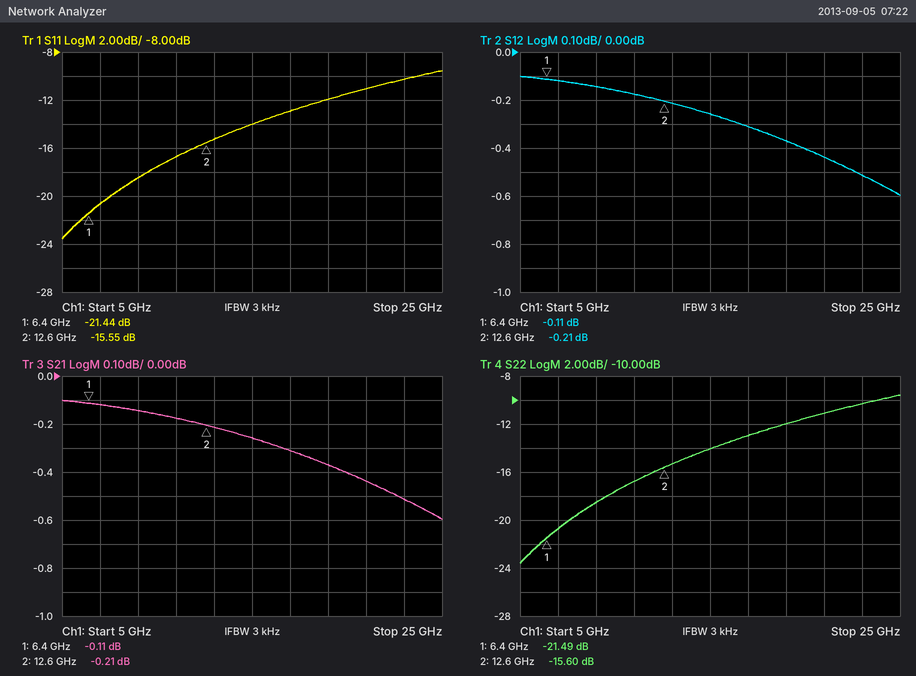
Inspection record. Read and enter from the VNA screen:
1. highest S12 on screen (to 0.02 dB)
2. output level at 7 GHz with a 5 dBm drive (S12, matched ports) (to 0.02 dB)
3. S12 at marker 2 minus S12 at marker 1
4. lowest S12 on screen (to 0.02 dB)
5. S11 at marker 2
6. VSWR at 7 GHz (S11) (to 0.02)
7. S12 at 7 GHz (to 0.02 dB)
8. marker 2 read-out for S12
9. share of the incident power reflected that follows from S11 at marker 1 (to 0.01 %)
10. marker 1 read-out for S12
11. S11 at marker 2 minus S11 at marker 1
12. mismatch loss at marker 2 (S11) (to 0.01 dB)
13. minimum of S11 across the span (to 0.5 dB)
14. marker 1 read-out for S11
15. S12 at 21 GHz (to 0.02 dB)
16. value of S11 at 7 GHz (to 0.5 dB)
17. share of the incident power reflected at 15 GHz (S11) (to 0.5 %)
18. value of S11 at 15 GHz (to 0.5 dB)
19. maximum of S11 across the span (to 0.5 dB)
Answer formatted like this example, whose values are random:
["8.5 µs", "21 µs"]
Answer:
["-0.10 dB", "4.88 dBm", "-0.10 dB", "-0.60 dB", "-15.55 dB", "1.20", "-0.12 dB", "-0.21 dB", "0.72 %", "-0.11 dB", "5.89 dB", "0.12 dB", "-23.5 dB", "-21.44 dB", "-0.44 dB", "-20.5 dB", "4.0 %", "-14.0 dB", "-9.5 dB"]
